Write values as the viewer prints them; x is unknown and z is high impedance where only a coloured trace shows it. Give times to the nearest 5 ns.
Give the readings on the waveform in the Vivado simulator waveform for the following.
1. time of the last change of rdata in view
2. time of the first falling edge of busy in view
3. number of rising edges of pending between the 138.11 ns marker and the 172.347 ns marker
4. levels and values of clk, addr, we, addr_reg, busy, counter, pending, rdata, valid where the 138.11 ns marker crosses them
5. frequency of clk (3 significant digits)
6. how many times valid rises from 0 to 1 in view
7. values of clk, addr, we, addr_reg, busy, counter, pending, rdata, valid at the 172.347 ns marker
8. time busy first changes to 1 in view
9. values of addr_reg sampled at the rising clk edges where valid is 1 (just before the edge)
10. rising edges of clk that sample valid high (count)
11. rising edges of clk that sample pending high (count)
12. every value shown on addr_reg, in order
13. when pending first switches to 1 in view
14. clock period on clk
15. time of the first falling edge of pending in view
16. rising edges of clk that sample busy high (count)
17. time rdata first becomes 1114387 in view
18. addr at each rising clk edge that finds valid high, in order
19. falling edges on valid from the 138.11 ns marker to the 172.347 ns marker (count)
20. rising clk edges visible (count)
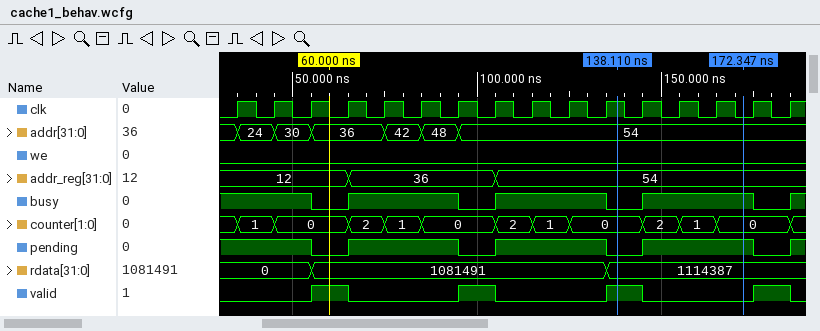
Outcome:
135 ns
55 ns
1
clk=1, addr=54, we=0, addr_reg=54, busy=0, counter=0, pending=0, rdata=1114387, valid=1
100 MHz
4
clk=0, addr=54, we=0, addr_reg=54, busy=1, counter=0, pending=1, rdata=1114387, valid=0
65 ns
12, 36, 54, 54
4
12
12, 36, 54
65 ns
10 ns
55 ns
12
135 ns
36, 54, 54, 54
1
16
